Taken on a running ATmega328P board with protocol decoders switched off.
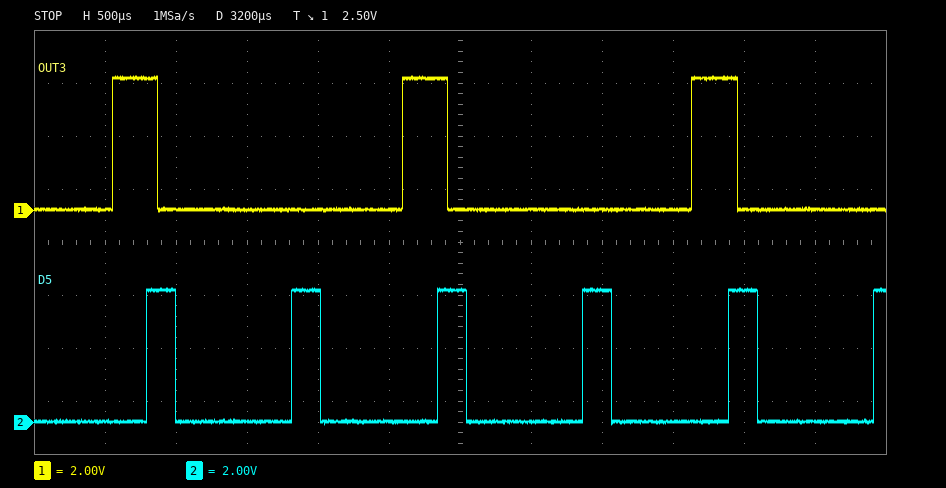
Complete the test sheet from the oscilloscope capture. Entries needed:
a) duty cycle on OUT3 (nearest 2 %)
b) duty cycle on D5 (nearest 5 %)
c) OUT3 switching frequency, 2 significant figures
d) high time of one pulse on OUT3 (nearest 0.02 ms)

16 %
20 %
490 Hz
0.32 ms
